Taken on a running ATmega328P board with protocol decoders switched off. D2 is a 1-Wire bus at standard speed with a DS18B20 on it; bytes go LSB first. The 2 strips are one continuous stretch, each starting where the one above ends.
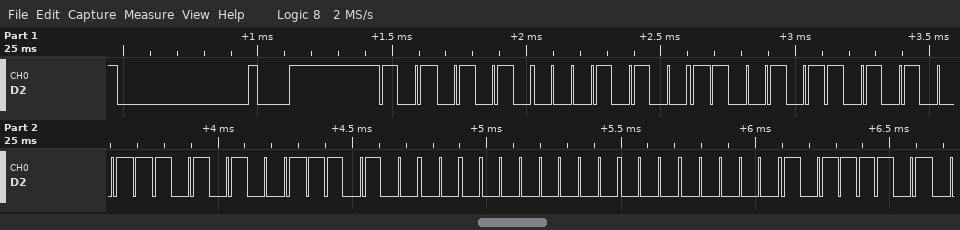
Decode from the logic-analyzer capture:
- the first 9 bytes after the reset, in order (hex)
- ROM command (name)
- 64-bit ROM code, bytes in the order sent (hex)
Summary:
55 28 D3 CA 95 0B 00 00 BD
Match ROM
28 D3 CA 95 0B 00 00 BD
